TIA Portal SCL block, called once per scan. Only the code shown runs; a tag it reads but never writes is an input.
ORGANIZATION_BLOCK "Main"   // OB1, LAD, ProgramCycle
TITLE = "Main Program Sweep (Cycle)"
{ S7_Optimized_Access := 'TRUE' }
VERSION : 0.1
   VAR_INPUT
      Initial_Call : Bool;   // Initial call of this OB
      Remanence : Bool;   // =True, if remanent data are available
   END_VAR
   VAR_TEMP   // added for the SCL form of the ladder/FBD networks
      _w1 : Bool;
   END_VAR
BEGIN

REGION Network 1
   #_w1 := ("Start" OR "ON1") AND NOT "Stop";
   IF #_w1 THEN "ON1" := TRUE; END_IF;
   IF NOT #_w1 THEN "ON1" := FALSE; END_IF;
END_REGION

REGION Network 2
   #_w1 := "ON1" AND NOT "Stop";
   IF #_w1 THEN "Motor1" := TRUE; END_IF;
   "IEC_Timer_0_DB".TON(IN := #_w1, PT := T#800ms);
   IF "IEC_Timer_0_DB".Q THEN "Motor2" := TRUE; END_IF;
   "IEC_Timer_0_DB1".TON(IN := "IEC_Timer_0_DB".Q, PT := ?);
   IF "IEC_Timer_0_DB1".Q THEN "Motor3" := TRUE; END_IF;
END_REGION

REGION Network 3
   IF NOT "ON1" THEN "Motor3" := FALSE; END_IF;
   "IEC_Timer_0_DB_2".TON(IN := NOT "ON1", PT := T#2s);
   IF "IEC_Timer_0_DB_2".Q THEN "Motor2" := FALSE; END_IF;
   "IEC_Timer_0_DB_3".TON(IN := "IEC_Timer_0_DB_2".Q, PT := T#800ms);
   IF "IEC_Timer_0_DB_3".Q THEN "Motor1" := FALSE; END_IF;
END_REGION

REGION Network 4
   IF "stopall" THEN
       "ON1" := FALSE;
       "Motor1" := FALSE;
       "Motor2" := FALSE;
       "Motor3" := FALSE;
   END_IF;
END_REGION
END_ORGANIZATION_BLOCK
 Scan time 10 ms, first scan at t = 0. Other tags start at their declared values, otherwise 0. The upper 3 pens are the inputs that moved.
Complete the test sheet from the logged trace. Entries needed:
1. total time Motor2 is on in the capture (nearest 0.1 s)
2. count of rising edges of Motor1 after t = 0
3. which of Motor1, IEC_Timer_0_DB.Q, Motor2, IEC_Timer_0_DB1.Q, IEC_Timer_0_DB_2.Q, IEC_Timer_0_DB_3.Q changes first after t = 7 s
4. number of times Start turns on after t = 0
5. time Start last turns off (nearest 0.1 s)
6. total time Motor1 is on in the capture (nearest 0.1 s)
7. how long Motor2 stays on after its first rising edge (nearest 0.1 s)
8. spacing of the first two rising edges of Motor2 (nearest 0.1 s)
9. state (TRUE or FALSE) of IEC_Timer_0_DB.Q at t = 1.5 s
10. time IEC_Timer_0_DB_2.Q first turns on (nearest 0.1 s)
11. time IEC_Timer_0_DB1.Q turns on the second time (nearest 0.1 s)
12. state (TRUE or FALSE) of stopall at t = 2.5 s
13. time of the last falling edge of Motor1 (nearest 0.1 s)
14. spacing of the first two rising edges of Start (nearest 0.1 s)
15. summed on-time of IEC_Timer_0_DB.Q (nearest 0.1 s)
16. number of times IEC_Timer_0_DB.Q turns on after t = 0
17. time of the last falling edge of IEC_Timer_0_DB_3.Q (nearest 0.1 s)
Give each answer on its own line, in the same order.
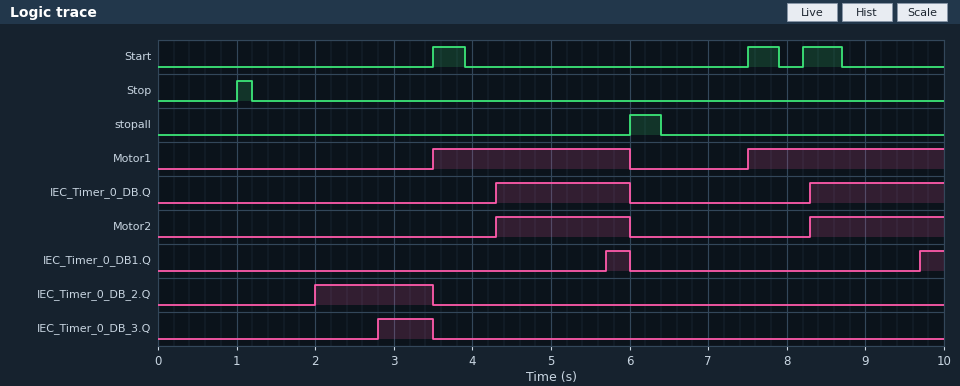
3.4 s
2
Motor1
3
8.7 s
5.0 s
1.7 s
4.0 s
FALSE
2.0 s
9.7 s
FALSE
6.0 s
4.0 s
3.4 s
2
3.5 s
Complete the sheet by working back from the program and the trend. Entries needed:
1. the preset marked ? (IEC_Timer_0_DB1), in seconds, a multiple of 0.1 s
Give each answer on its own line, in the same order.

1.4 s
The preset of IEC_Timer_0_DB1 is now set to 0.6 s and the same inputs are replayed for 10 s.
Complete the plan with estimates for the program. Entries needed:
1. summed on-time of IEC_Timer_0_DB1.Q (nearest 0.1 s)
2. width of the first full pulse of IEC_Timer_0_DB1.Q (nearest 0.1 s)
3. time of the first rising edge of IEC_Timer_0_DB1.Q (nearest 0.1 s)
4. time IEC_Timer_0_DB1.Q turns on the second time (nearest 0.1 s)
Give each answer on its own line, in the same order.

2.2 s
1.1 s
4.9 s
8.9 s
